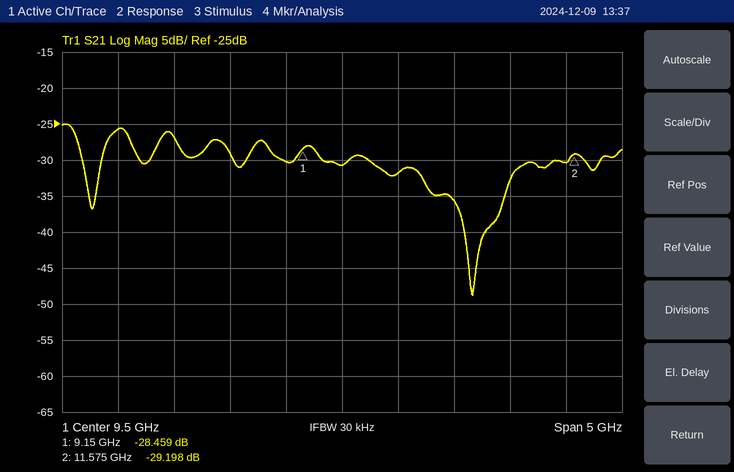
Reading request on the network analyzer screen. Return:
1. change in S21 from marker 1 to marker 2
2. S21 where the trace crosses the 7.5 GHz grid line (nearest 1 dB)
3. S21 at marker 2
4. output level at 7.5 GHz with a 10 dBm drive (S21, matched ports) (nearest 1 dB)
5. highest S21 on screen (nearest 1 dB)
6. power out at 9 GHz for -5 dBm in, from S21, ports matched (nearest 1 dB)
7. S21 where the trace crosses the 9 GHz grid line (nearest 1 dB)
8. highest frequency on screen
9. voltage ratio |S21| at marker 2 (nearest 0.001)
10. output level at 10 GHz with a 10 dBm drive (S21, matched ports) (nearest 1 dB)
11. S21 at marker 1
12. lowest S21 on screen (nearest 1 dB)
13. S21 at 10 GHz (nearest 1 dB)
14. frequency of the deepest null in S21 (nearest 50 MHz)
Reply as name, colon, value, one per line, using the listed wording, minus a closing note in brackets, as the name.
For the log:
change in S21 from marker 1 to marker 2: -0.739 dB
S21 where the trace crosses the 7.5 GHz grid line: -26 dB
S21 at marker 2: -29.198 dB
output level at 7.5 GHz with a 10 dBm drive (S21, matched ports): -16 dBm
highest S21 on screen: -25 dB
power out at 9 GHz for -5 dBm in, from S21, ports matched: -35 dBm
S21 where the trace crosses the 9 GHz grid line: -30 dB
highest frequency on screen: 12 GHz
voltage ratio |S21| at marker 2: 0.035
output level at 10 GHz with a 10 dBm drive (S21, matched ports): -22 dBm
S21 at marker 1: -28.459 dB
lowest S21 on screen: -49 dB
S21 at 10 GHz: -32 dB
frequency of the deepest null in S21: 10.65 GHz
